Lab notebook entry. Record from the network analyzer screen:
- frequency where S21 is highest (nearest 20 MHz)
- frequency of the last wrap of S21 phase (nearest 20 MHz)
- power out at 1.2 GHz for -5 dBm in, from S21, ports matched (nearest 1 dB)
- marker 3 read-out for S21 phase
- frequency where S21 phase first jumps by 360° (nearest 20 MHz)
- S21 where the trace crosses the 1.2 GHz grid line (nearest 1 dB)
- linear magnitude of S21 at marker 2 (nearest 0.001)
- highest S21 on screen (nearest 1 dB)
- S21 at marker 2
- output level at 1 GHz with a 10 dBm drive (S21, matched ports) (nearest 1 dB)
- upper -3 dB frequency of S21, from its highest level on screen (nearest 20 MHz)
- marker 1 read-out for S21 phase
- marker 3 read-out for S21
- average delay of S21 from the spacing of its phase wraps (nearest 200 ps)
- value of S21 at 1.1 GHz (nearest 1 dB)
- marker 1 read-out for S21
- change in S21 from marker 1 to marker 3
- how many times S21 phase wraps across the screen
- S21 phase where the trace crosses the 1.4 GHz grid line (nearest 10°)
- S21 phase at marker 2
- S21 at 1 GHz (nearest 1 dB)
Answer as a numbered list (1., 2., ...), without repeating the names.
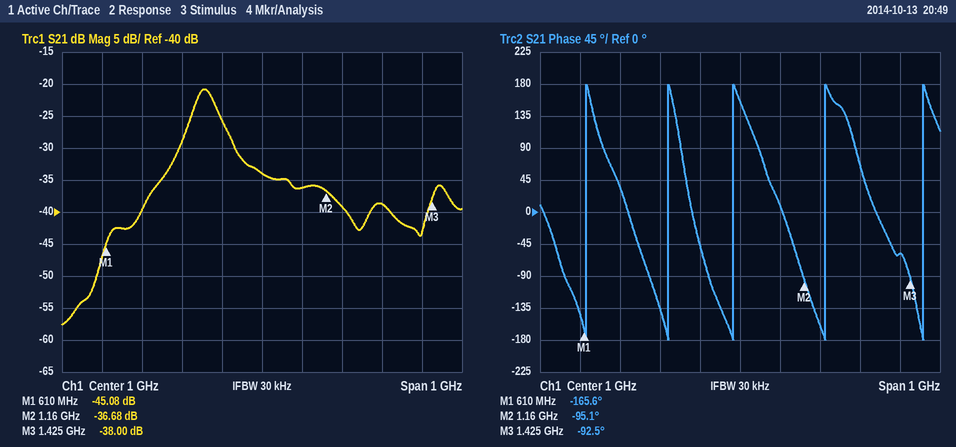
1. 860 MHz
2. 1.46 GHz
3. -44 dBm
4. -92.5°
5. 620 MHz
6. -39 dB
7. 0.015
8. -21 dB
9. -36.68 dB
10. -24 dBm
11. 880 MHz
12. -165.6°
13. -38.00 dB
14. 4.8 ns
15. -36 dB
16. -45.08 dB
17. 7.08 dB
18. 5
19. -60°
20. -95.1°
21. -34 dB
